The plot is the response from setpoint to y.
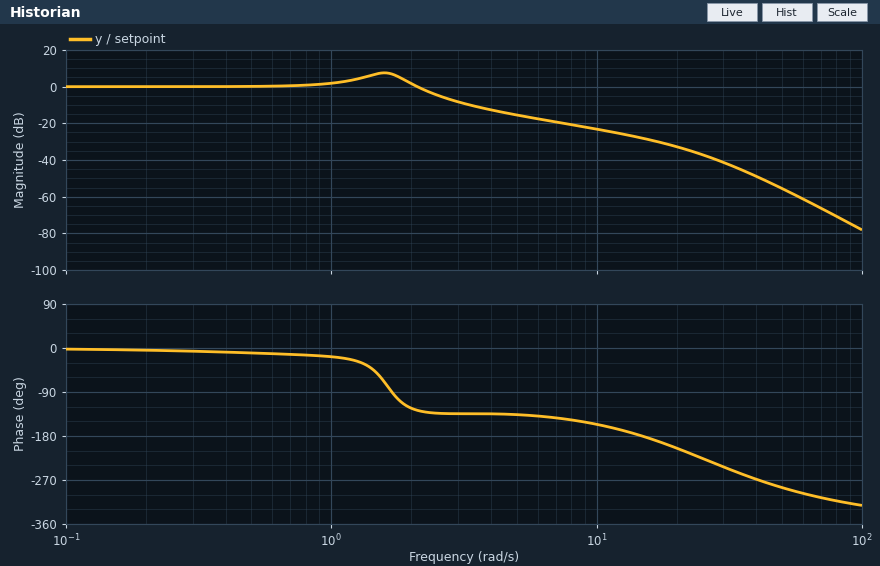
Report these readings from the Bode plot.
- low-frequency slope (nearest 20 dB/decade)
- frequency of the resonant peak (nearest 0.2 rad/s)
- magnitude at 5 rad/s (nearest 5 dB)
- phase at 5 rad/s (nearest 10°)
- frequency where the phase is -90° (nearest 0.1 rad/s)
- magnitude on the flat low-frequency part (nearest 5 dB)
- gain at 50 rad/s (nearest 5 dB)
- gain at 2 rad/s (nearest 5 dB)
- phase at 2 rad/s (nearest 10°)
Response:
0 dB/decade
1.6 rad/s
-15 dB
-140°
1.7 rad/s
0 dB
-55 dB
0 dB
-120°
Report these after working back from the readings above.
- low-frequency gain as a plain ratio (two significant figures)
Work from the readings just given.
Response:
1.0
